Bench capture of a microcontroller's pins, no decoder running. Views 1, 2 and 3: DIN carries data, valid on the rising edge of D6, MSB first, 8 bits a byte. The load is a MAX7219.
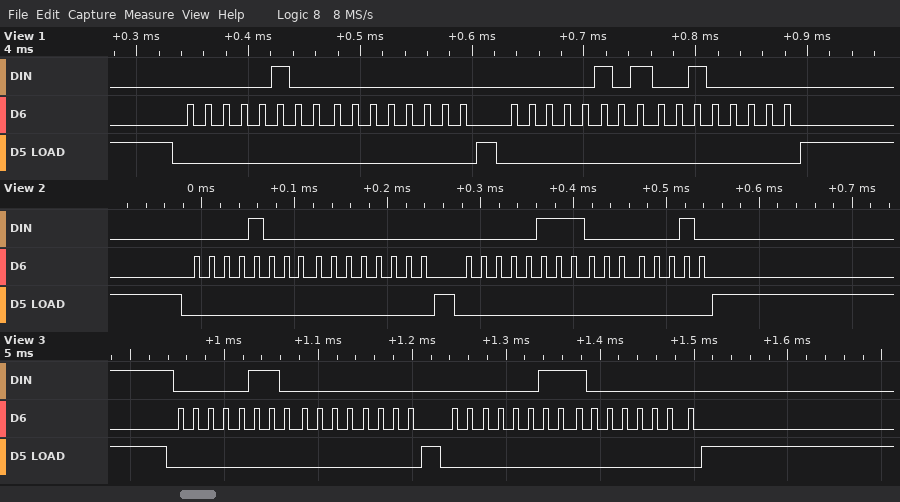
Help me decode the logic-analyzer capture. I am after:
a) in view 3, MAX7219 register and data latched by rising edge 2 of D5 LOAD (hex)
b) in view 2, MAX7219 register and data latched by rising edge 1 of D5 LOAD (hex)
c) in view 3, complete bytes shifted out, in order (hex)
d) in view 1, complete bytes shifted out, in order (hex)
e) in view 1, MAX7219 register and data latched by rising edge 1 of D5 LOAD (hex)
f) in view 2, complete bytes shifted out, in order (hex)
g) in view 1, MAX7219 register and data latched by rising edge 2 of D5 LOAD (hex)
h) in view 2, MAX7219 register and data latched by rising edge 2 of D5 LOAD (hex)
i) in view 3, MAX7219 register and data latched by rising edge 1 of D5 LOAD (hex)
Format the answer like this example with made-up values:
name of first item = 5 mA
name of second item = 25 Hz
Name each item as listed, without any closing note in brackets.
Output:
in view 3, MAX7219 register and data latched by rising edge 2 of D5 LOAD = register 0x3, data 0x80
in view 2, MAX7219 register and data latched by rising edge 1 of D5 LOAD = register 0x8, data 0x00
in view 3, complete bytes shifted out, in order = 06 00 03 80
in view 1, complete bytes shifted out, in order = 04 00 05 20
in view 1, MAX7219 register and data latched by rising edge 1 of D5 LOAD = register 0x4, data 0x00
in view 2, complete bytes shifted out, in order = 08 00 07 02
in view 1, MAX7219 register and data latched by rising edge 2 of D5 LOAD = register 0x5, data 0x20
in view 2, MAX7219 register and data latched by rising edge 2 of D5 LOAD = register 0x7, data 0x02
in view 3, MAX7219 register and data latched by rising edge 1 of D5 LOAD = register 0x6, data 0x00
